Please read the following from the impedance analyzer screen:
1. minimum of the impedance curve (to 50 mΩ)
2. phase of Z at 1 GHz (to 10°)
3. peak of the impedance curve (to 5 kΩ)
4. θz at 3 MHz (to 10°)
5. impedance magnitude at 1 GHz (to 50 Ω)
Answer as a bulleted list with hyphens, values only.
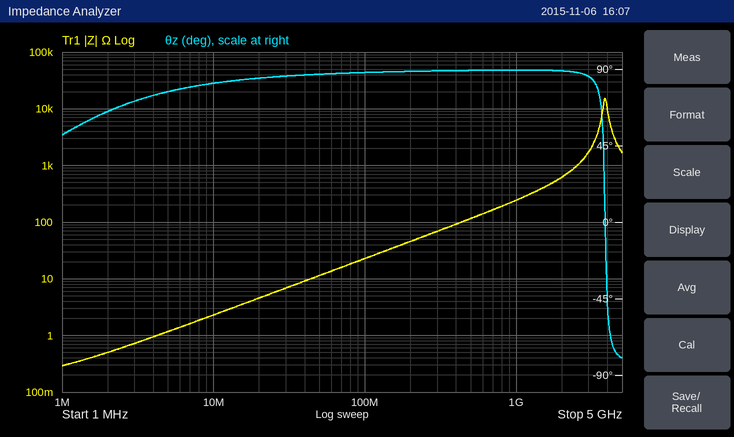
- 300 mΩ
- 90°
- 15 kΩ
- 70°
- 250 Ω
